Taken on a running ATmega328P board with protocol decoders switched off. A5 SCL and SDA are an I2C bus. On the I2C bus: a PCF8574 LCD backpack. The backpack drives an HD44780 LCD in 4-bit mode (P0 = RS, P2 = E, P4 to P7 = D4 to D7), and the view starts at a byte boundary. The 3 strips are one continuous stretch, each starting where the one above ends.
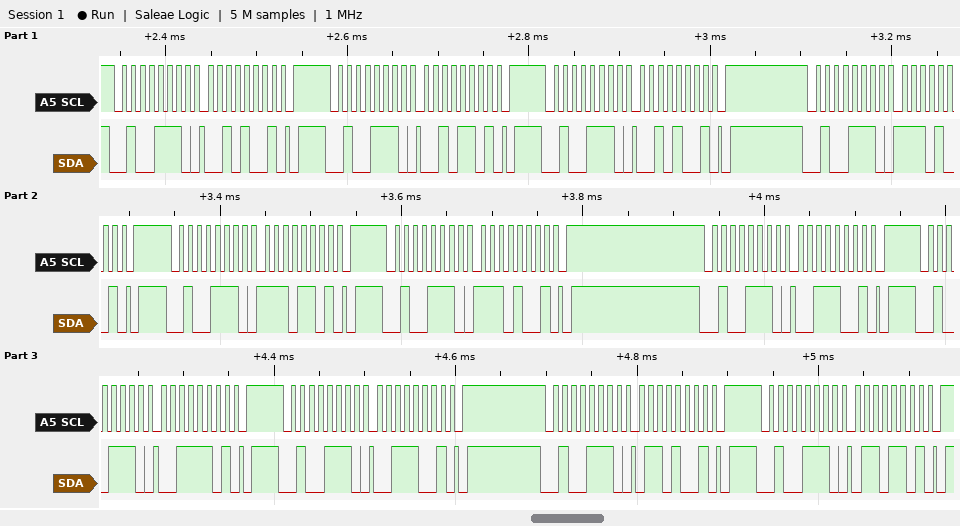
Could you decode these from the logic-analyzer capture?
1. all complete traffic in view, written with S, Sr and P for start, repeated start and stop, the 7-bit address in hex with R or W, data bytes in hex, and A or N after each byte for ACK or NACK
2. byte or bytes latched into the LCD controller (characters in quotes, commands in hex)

S 27W A 29 A P S 27W A 2D A P S 27W A 29 A P S 27W A E9 A P S 27W A ED A P S 27W A E9 A P S 27W A 39 A P S 27W A 3D A P S 27W A 39 A P S 27W A 69 A P S 27W A 6D A P
'.'
